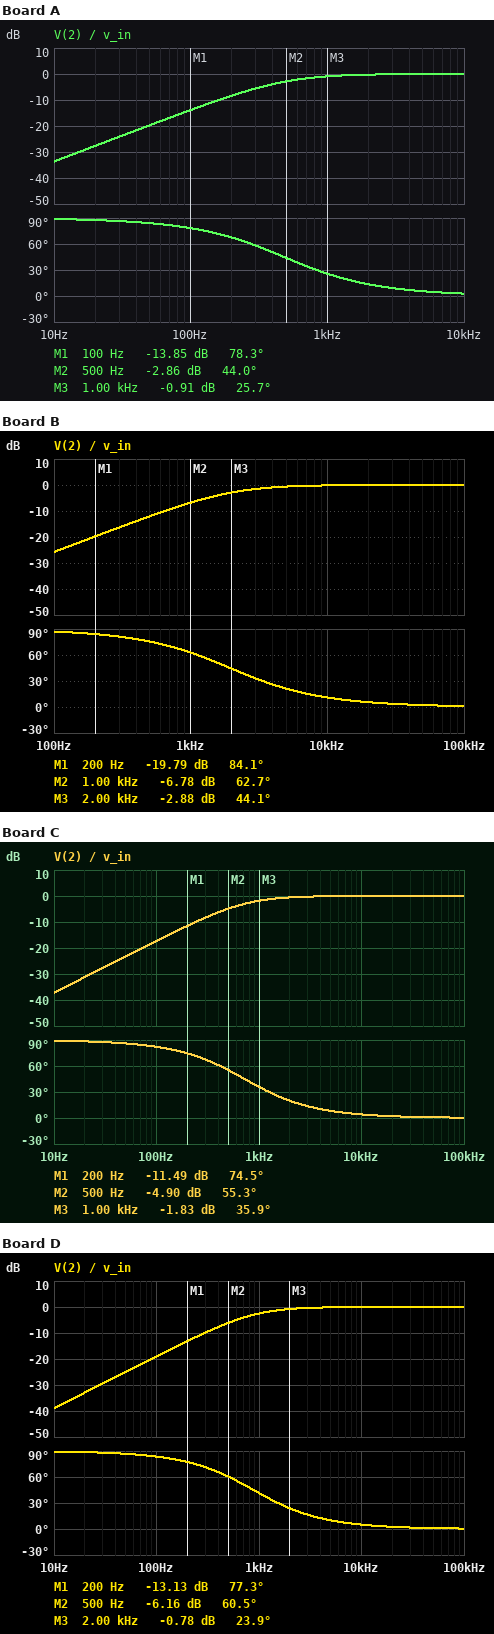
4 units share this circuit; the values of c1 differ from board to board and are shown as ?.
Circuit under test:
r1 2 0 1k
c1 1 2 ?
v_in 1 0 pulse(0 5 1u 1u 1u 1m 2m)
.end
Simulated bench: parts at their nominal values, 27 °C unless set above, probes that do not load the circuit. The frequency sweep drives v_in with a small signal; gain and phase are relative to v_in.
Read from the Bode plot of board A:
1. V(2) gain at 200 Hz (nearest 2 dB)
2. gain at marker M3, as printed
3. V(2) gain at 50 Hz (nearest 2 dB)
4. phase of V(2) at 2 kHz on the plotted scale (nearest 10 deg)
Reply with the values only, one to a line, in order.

-8 dB
-0.91 dB
-20 dB
10 deg
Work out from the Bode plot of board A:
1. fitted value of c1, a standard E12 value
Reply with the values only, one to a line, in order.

330 nF
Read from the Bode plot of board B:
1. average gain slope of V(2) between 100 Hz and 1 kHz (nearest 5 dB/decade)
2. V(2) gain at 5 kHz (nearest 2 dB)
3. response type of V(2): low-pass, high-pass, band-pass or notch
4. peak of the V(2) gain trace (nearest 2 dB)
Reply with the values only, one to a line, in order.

20 dB/decade
0 dB
high-pass
0 dB
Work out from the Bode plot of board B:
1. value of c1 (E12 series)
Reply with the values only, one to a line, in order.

82 nF
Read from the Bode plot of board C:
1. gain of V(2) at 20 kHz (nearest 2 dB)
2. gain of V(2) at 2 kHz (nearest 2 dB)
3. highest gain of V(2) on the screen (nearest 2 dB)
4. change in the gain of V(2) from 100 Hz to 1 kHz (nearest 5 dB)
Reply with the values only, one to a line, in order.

0 dB
0 dB
0 dB
15 dB
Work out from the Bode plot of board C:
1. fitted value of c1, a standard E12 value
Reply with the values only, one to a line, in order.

220 nF
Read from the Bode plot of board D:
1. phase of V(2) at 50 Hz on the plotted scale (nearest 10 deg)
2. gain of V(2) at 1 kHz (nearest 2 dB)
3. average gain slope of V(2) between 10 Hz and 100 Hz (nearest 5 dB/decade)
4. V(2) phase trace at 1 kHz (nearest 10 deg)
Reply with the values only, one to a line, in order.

90 deg
-2 dB
20 dB/decade
40 deg
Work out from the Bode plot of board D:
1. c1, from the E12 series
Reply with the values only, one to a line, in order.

180 nF
